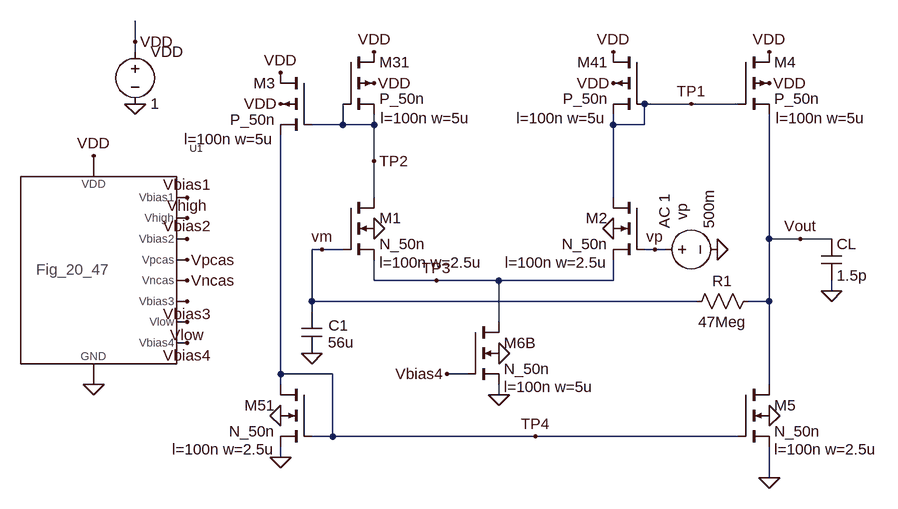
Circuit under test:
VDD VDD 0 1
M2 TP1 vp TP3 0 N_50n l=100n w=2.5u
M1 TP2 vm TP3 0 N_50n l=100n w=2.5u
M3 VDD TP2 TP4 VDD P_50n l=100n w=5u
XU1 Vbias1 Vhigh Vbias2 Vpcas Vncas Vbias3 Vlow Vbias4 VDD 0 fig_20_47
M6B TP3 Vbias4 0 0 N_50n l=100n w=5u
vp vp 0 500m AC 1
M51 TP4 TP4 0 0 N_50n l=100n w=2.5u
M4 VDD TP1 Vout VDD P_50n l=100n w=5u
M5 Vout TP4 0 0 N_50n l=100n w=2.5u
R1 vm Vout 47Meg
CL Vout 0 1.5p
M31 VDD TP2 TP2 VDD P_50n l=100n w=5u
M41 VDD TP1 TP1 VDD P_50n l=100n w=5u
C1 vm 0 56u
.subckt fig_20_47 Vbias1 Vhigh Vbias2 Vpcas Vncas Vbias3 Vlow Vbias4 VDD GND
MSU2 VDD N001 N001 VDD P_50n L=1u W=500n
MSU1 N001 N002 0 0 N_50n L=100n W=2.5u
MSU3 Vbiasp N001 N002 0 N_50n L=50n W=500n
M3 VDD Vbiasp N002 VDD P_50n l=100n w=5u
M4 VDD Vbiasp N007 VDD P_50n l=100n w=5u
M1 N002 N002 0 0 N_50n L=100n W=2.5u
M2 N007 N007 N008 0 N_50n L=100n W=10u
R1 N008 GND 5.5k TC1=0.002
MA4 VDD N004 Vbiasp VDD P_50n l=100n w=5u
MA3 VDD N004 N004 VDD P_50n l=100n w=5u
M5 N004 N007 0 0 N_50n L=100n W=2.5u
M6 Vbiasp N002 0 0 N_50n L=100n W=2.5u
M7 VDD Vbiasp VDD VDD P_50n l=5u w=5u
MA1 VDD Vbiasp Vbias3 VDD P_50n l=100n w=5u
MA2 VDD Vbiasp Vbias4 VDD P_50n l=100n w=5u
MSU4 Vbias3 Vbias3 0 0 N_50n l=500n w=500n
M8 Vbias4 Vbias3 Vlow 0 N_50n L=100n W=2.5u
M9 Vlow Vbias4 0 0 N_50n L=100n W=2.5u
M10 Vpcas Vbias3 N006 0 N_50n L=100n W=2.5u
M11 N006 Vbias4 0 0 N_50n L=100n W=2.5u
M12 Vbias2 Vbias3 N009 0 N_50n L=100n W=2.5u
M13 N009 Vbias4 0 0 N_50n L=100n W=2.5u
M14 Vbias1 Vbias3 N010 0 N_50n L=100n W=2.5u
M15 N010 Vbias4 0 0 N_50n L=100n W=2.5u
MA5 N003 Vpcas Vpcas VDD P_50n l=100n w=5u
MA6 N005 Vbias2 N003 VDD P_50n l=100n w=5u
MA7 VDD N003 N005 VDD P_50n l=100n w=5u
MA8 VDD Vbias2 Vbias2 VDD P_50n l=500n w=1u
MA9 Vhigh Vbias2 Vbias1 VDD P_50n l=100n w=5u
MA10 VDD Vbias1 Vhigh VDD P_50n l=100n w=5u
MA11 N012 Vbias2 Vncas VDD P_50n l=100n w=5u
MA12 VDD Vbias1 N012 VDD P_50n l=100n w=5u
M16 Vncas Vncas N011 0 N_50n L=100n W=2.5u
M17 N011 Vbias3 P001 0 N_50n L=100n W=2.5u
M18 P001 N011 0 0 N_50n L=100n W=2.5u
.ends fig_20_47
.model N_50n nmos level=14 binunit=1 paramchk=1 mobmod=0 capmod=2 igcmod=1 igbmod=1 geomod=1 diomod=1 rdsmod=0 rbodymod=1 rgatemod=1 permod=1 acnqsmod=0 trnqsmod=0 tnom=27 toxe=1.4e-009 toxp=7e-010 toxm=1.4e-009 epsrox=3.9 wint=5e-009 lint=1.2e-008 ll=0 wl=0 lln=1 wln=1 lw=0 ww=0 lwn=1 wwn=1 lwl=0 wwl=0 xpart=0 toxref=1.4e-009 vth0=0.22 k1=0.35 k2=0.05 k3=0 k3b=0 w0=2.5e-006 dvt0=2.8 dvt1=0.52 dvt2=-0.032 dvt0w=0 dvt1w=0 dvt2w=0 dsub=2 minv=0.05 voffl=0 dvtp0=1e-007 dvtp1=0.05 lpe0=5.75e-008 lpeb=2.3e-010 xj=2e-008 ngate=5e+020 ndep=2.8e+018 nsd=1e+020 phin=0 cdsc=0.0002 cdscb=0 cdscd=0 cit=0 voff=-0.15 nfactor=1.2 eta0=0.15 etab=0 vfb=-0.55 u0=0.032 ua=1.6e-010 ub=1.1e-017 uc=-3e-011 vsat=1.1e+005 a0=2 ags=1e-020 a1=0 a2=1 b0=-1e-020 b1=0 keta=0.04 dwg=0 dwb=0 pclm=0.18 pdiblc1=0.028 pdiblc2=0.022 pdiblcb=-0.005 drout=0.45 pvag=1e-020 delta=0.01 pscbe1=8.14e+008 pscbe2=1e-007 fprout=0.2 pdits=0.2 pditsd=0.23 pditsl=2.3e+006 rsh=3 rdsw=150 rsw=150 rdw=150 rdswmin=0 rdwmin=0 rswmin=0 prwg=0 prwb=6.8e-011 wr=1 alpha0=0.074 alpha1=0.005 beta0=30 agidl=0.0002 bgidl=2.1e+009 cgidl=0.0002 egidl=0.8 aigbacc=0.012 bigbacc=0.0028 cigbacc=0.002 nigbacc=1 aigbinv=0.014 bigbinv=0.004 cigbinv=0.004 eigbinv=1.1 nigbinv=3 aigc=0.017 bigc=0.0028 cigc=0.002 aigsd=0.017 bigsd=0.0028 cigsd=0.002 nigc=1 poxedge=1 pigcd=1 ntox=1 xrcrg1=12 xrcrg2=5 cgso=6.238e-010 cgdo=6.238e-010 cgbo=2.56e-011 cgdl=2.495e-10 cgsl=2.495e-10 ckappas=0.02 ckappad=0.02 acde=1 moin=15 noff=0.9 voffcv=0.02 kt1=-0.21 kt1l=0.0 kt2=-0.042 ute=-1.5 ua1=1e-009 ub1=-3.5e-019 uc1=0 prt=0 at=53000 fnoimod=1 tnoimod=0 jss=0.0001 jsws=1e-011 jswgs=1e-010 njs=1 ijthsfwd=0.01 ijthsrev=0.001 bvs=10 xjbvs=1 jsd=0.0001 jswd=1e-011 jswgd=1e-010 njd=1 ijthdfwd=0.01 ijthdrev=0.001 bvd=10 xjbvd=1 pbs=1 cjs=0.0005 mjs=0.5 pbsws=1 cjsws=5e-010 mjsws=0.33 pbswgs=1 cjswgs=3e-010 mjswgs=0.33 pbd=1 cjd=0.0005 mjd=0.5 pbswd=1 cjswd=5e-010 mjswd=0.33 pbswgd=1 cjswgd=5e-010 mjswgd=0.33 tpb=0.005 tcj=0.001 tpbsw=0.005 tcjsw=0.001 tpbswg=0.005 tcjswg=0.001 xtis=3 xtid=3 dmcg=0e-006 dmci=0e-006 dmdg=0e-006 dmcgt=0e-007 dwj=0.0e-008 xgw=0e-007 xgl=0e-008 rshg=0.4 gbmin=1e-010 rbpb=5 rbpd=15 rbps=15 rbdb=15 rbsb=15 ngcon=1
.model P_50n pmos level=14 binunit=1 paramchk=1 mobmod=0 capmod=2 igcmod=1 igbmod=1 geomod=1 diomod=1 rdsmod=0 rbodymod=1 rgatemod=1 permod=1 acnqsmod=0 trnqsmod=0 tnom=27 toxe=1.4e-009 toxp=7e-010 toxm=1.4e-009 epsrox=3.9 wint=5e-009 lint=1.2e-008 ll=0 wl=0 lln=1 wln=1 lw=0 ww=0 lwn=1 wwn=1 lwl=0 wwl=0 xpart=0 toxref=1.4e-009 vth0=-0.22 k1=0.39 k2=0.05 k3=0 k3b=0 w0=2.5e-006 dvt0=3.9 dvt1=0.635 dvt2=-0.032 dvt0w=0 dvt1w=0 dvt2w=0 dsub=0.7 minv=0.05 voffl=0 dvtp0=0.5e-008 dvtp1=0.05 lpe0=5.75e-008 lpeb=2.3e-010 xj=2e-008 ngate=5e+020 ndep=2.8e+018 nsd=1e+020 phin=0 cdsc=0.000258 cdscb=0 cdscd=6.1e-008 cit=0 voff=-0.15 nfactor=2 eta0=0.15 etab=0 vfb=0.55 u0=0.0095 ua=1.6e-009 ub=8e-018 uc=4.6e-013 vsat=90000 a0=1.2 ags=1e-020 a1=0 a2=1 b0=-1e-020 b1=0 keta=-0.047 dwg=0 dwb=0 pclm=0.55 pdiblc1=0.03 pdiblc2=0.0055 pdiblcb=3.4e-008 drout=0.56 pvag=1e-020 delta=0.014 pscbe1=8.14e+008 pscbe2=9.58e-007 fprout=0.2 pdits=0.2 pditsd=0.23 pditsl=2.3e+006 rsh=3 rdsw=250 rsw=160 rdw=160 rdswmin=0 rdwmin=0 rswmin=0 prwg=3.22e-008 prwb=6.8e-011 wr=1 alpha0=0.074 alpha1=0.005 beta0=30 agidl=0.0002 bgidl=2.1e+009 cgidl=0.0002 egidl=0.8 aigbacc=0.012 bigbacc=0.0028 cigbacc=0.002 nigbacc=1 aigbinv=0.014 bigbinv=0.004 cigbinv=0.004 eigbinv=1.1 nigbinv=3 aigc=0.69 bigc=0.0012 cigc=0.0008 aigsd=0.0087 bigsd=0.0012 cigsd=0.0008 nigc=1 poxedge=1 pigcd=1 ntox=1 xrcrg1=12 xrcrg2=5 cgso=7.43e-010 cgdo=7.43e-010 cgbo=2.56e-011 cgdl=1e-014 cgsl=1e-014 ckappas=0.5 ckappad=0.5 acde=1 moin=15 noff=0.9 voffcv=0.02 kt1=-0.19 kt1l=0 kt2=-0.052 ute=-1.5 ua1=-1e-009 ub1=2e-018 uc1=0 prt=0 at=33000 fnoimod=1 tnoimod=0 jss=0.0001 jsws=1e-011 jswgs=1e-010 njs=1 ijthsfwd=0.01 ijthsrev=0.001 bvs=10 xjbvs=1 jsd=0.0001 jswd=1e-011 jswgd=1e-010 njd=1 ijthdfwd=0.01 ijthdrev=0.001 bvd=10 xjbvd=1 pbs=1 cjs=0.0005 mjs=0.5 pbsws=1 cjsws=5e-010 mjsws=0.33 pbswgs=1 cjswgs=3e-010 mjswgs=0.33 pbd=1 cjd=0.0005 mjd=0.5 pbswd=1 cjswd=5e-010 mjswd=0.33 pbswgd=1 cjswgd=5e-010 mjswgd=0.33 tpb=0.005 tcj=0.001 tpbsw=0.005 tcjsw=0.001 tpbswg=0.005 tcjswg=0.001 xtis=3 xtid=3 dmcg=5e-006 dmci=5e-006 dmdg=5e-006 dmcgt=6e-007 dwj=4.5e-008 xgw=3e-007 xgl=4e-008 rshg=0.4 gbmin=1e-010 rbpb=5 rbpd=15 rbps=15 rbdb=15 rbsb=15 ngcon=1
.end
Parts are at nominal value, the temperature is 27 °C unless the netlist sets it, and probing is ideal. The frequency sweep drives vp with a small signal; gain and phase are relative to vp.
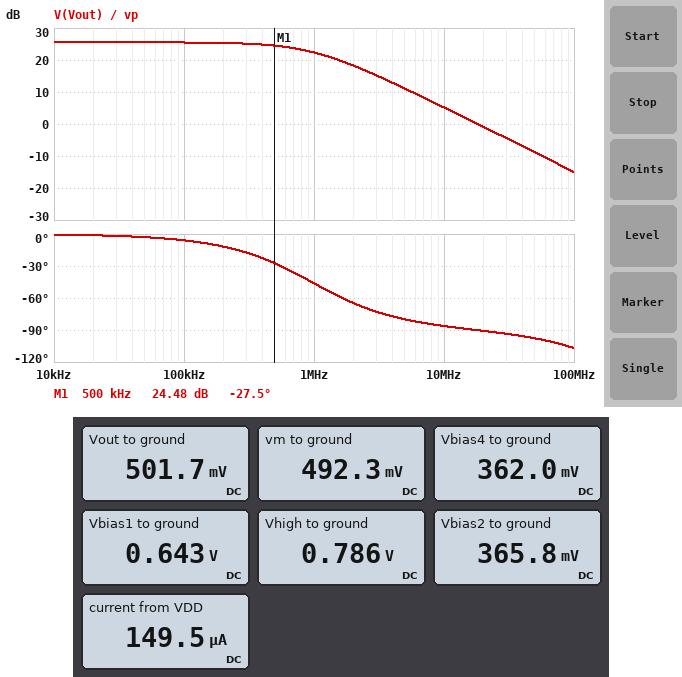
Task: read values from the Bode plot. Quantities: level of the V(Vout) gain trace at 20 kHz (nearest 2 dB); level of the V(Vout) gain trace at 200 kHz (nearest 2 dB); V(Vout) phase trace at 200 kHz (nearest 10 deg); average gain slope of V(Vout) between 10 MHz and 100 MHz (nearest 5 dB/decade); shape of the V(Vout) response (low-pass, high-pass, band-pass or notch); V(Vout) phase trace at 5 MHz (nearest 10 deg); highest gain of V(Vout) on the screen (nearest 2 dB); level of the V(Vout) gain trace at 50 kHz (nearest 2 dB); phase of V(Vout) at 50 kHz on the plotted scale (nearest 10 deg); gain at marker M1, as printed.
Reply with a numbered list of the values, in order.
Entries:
1. 26 dB
2. 26 dB
3. -10 deg
4. -20 dB/decade
5. low-pass
6. -80 deg
7. 26 dB
8. 26 dB
9. 0 deg
10. 24.48 dB
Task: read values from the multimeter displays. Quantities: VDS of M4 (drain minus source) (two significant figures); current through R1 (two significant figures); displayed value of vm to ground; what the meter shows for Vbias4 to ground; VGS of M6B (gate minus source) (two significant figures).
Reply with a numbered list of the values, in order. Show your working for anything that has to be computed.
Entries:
1. 1 V - 501.7 mV = 500 mV
2. (501.7 mV - 492.3 mV) / 47 MΩ = 200 pA
3. 492.3 mV
4. 362.0 mV
5. 362 mV = 360 mV
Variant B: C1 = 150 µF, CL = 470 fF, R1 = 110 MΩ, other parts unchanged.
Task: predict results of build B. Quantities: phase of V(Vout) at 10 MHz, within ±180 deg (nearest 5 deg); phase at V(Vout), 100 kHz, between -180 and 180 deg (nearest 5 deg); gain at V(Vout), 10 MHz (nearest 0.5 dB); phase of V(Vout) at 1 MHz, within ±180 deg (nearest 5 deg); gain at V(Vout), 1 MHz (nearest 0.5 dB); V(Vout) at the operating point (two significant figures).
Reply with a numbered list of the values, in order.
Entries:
1. -75 deg
2. 0 deg
3. 14.5 dB
4. -20 deg
5. 25.0 dB
6. 510 mV
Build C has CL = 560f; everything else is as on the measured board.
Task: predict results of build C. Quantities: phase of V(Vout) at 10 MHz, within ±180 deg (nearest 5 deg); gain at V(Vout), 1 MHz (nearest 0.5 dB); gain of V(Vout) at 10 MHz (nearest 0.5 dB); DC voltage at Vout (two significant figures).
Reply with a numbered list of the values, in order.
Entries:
1. -80 deg
2. 25.0 dB
3. 13.0 dB
4. 500 mV
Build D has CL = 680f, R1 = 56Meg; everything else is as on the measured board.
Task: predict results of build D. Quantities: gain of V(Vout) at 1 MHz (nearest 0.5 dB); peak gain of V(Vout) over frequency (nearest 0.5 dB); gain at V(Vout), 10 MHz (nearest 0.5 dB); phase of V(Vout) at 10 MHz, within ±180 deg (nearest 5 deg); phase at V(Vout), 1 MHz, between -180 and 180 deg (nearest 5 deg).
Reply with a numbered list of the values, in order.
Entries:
1. 24.5 dB
2. 25.5 dB
3. 11.5 dB
4. -80 deg
5. -25 deg
